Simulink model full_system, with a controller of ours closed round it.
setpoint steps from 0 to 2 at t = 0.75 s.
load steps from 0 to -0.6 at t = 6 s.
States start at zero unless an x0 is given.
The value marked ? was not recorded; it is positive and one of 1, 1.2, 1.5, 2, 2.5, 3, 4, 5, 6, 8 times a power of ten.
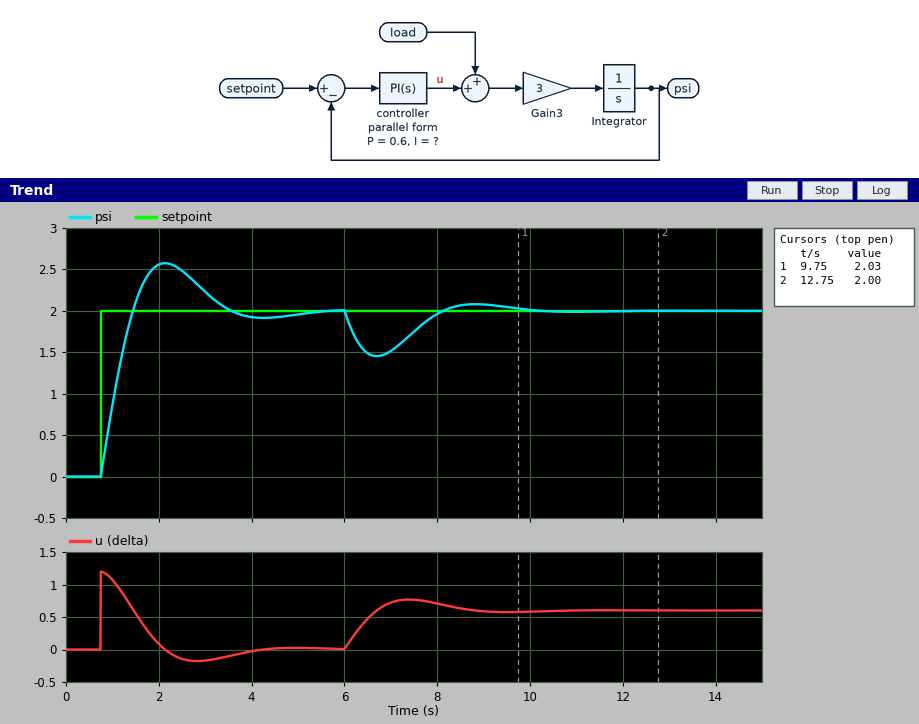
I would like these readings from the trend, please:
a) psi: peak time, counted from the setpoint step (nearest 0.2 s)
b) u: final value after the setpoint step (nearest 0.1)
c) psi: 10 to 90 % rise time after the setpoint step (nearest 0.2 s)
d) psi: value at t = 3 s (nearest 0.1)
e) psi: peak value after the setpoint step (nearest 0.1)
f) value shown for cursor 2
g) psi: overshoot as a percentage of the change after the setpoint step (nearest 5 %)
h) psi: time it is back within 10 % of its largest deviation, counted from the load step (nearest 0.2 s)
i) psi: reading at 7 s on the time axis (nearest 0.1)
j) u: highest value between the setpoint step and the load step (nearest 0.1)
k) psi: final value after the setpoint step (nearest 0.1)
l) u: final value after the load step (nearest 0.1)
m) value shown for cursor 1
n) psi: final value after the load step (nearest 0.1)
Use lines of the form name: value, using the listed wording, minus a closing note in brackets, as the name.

psi: peak time, counted from the setpoint step: 1.4 s
u: final value after the setpoint step: 0.0
psi: 10 to 90 % rise time after the setpoint step: 0.6 s
psi: value at t = 3 s: 2.2
psi: peak value after the setpoint step: 2.6
value shown for cursor 2: 2.00
psi: overshoot as a percentage of the change after the setpoint step: 30 %
psi: time it is back within 10 % of its largest deviation, counted from the load step: 3.4 s
psi: reading at 7 s on the time axis: 1.5
u: highest value between the setpoint step and the load step: 1.2
psi: final value after the setpoint step: 2.0
u: final value after the load step: 0.6
value shown for cursor 1: 2.03
psi: final value after the load step: 2.0
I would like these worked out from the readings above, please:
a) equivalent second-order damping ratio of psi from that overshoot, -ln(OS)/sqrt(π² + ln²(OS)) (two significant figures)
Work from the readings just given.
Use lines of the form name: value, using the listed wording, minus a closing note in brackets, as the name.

equivalent second-order damping ratio of psi from that overshoot, -ln(OS)/sqrt(π² + ln²(OS)): 0.36
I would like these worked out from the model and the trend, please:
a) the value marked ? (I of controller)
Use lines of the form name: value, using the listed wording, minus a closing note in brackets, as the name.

the value marked ?: 1
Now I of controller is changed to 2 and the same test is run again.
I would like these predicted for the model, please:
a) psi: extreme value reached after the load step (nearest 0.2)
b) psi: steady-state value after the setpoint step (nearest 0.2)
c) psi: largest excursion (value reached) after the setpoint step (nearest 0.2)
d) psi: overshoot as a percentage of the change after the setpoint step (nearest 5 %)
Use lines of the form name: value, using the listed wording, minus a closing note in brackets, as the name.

psi: extreme value reached after the load step: 1.6
psi: steady-state value after the setpoint step: 2.0
psi: largest excursion (value reached) after the setpoint step: 2.8
psi: overshoot as a percentage of the change after the setpoint step: 40 %
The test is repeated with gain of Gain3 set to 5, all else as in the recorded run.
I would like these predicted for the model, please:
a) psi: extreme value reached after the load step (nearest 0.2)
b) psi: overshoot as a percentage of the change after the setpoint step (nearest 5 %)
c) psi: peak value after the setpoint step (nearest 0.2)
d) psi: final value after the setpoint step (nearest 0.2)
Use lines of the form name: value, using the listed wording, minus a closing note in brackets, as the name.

psi: extreme value reached after the load step: 1.4
psi: overshoot as a percentage of the change after the setpoint step: 20 %
psi: peak value after the setpoint step: 2.4
psi: final value after the setpoint step: 2.0
